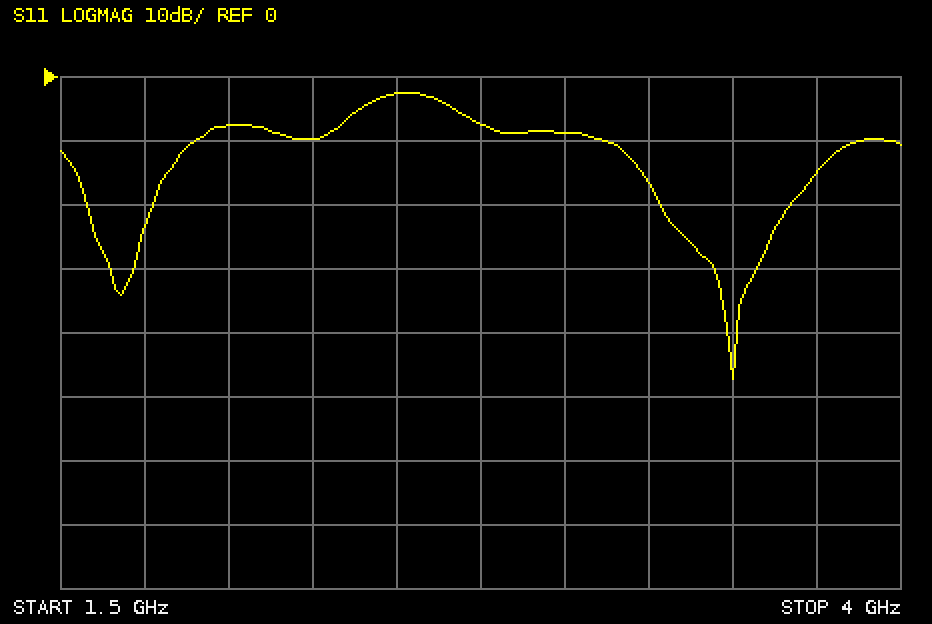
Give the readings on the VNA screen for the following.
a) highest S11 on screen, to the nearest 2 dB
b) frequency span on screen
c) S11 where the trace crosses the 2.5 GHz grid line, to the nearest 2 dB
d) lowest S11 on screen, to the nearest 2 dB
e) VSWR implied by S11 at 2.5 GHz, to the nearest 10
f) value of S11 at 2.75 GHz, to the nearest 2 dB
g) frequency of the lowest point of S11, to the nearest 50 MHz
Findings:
-2 dB
2.5 GHz
-2 dB
-48 dB
10
-8 dB
3.50 GHz
